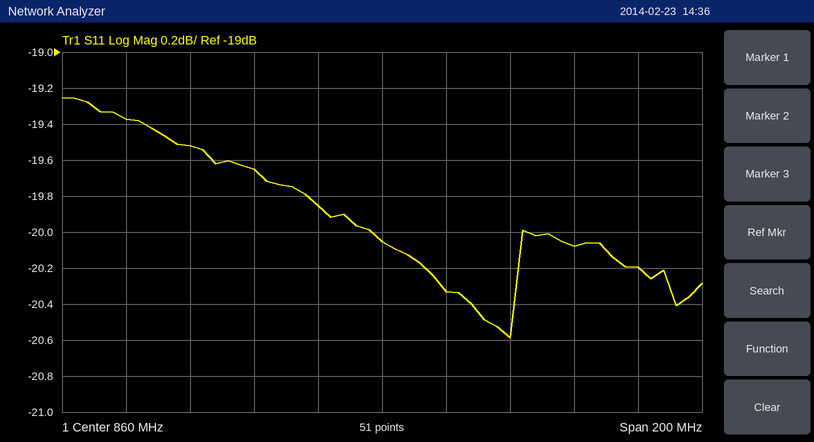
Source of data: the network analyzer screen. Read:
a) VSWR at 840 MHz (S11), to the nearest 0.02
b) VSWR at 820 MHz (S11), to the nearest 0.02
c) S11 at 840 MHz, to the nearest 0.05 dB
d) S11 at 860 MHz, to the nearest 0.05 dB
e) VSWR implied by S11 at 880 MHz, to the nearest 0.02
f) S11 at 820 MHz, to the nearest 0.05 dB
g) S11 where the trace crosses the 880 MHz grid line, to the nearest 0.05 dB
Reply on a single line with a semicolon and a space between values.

1.22; 1.24; -19.85 dB; -20.05 dB; 1.22; -19.65 dB; -20.35 dB
